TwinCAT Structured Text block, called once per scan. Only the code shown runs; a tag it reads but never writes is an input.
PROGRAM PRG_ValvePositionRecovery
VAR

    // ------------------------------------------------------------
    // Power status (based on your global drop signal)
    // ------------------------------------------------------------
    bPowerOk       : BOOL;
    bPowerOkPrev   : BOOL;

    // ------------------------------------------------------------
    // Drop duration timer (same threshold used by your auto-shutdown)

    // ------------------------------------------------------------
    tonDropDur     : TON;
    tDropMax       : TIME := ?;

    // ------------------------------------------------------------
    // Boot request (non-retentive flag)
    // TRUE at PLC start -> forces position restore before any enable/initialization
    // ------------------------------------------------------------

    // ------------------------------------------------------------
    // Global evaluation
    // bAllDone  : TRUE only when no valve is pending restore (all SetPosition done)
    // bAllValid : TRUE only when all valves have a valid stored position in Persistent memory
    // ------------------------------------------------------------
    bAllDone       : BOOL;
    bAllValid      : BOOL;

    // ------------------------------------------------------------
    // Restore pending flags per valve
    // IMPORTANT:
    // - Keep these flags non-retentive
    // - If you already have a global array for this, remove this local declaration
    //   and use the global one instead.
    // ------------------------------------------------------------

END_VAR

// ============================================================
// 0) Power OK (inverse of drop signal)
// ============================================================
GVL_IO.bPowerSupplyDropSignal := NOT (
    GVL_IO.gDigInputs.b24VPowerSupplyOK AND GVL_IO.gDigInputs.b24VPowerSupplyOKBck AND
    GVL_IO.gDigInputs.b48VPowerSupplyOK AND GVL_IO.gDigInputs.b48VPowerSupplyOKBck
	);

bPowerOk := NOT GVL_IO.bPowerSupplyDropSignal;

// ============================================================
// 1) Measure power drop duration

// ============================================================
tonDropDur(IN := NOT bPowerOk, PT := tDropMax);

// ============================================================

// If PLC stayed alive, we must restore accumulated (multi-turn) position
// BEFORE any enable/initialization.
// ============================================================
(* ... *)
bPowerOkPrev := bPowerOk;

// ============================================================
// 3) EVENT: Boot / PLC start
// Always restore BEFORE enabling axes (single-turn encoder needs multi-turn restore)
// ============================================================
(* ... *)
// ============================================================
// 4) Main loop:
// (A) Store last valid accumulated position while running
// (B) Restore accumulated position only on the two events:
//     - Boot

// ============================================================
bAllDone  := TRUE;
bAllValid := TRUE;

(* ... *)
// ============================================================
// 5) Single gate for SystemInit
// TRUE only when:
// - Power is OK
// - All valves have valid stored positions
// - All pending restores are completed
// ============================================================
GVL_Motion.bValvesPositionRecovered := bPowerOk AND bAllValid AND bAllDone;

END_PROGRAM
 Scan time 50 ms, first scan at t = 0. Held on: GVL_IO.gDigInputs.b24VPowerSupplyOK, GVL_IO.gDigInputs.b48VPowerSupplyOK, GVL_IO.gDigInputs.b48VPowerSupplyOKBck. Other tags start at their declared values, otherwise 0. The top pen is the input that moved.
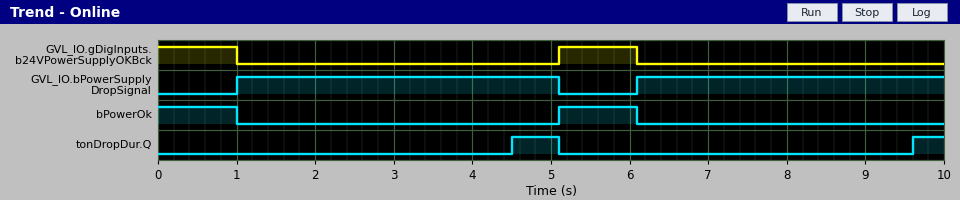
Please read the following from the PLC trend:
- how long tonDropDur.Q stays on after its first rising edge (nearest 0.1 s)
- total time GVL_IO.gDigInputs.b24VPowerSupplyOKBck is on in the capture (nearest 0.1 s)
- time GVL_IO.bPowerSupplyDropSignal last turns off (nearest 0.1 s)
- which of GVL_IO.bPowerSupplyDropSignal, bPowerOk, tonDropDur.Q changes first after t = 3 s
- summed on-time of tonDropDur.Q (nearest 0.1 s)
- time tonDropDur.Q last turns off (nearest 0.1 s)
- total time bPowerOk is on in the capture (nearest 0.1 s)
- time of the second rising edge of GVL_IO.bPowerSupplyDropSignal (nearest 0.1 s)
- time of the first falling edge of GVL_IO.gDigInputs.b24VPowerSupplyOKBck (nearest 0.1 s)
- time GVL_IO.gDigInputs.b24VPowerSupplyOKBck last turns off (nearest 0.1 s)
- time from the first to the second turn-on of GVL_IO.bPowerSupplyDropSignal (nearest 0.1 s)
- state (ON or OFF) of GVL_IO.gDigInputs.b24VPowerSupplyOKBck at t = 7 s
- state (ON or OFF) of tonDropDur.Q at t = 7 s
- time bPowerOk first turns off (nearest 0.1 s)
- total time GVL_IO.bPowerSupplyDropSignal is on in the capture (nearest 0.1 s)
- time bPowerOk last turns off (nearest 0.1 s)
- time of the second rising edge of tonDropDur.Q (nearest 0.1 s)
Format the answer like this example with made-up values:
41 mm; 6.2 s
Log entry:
0.6 s; 2.0 s; 5.1 s; tonDropDur.Q; 1.0 s; 5.1 s; 2.0 s; 6.1 s; 1.0 s; 6.1 s; 5.1 s; OFF; OFF; 1.0 s; 8.0 s; 6.1 s; 9.6 s
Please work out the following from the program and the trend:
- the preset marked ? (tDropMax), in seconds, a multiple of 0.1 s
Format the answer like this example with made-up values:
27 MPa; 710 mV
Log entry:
3.5 s
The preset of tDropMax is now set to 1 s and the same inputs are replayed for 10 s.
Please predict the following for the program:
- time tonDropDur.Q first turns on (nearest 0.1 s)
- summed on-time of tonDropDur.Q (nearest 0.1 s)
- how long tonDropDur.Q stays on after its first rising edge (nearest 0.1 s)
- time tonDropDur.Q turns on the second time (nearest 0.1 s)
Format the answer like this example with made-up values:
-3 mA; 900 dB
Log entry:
2.0 s; 6.0 s; 3.1 s; 7.1 s
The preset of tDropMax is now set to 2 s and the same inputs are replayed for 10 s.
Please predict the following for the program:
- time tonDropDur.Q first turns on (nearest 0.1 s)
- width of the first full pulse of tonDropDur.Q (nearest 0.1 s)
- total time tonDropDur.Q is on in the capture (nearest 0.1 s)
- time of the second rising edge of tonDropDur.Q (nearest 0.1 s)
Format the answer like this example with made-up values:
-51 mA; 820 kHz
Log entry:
3.0 s; 2.1 s; 4.0 s; 8.1 s
